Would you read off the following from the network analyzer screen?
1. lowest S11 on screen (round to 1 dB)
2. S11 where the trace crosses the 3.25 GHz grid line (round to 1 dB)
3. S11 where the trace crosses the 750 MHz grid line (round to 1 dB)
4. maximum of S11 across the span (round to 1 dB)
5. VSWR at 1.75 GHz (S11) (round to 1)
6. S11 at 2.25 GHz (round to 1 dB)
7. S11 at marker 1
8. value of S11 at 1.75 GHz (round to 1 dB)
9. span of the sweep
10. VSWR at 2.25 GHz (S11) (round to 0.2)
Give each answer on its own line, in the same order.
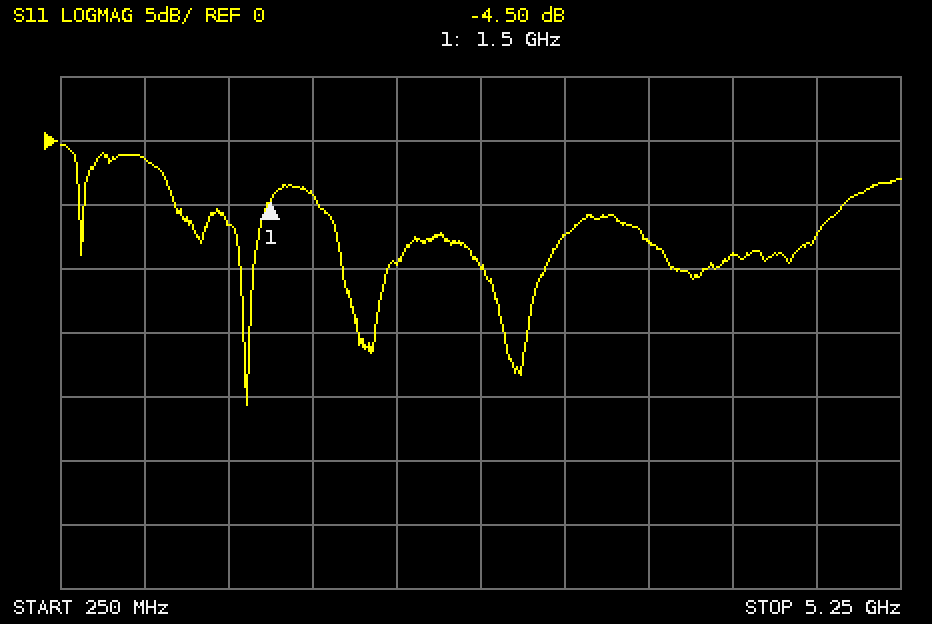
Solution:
-21 dB
-7 dB
-1 dB
0 dB
4
-10 dB
-4.50 dB
-4 dB
5 GHz
2.0
